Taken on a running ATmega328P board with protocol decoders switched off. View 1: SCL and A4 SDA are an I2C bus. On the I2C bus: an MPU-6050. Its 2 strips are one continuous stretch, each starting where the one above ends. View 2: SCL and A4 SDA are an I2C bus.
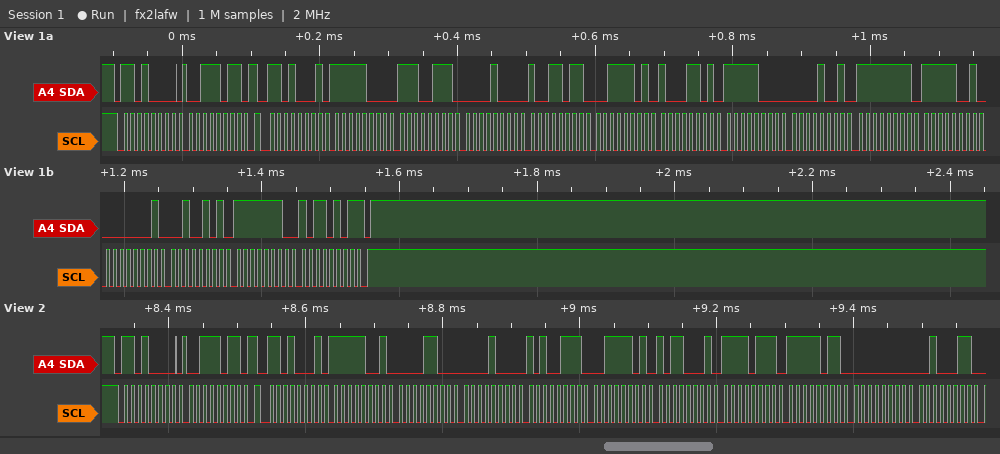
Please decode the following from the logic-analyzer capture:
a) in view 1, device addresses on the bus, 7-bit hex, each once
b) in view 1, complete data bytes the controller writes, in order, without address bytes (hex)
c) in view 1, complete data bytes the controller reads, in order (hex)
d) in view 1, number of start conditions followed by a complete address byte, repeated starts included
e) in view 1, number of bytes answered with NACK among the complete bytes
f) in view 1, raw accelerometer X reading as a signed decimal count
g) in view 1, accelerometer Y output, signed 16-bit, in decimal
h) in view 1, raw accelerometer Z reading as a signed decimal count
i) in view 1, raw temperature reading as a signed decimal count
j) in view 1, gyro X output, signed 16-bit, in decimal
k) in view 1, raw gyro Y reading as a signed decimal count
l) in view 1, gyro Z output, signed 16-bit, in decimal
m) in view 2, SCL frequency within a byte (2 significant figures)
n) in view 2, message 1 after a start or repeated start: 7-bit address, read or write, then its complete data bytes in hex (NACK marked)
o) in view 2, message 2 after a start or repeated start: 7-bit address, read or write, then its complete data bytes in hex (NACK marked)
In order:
0x68
3B
F8 E7 08 9B 3D 8D F8 09 FF F9 01 25 FE B5
2
1
-1817
2203
15757
-2039
-7
293
-331
100 kHz
0x68 write: 3B
0x68 read: F9 0C 08 A7 3D B1 F7 FB 00 23
